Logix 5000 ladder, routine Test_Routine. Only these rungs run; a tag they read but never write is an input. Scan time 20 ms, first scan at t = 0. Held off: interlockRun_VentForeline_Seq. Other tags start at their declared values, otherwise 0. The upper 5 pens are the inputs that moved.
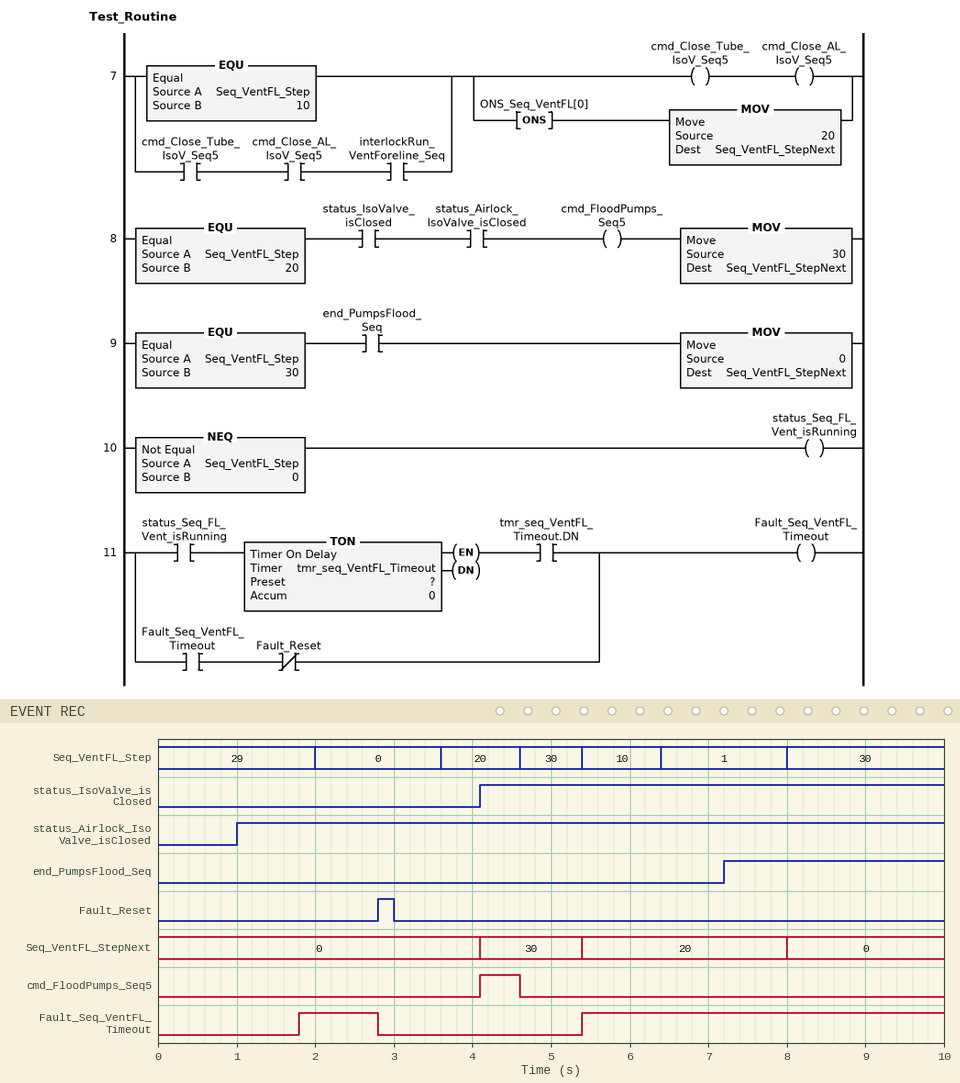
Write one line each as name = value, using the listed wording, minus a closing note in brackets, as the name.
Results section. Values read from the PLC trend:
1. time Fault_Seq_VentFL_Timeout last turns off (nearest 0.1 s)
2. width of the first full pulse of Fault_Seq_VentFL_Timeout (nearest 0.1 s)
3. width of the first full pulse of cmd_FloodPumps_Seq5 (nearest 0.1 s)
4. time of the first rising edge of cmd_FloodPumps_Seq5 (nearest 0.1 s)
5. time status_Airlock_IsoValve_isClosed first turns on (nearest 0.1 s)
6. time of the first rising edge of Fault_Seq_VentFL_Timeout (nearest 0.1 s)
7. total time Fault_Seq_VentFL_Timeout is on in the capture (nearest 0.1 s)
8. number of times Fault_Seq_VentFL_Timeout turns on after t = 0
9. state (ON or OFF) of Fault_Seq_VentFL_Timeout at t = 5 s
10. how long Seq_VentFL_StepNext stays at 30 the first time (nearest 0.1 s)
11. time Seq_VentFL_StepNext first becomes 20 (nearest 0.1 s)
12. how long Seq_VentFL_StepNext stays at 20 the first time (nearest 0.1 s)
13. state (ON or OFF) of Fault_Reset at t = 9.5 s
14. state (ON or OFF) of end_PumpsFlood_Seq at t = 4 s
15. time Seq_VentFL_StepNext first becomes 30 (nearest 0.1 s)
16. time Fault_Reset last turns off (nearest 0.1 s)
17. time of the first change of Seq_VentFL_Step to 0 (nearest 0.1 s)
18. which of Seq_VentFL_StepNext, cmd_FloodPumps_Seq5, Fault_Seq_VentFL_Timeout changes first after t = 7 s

time Fault_Seq_VentFL_Timeout last turns off = 2.8 s
width of the first full pulse of Fault_Seq_VentFL_Timeout = 1.0 s
width of the first full pulse of cmd_FloodPumps_Seq5 = 0.5 s
time of the first rising edge of cmd_FloodPumps_Seq5 = 4.1 s
time status_Airlock_IsoValve_isClosed first turns on = 1.0 s
time of the first rising edge of Fault_Seq_VentFL_Timeout = 1.8 s
total time Fault_Seq_VentFL_Timeout is on in the capture = 5.6 s
number of times Fault_Seq_VentFL_Timeout turns on after t = 0 = 2
state (ON or OFF) of Fault_Seq_VentFL_Timeout at t = 5 s = OFF
how long Seq_VentFL_StepNext stays at 30 the first time = 1.3 s
time Seq_VentFL_StepNext first becomes 20 = 5.4 s
how long Seq_VentFL_StepNext stays at 20 the first time = 2.6 s
state (ON or OFF) of Fault_Reset at t = 9.5 s = OFF
state (ON or OFF) of end_PumpsFlood_Seq at t = 4 s = OFF
time Seq_VentFL_StepNext first becomes 30 = 4.1 s
time Fault_Reset last turns off = 3.0 s
time of the first change of Seq_VentFL_Step to 0 = 2.0 s
which of Seq_VentFL_StepNext, cmd_FloodPumps_Seq5, Fault_Seq_VentFL_Timeout changes first after t = 7 s = Seq_VentFL_StepNext
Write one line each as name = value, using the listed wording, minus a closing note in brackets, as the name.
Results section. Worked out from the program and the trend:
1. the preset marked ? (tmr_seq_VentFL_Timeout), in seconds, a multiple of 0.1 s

the preset marked ? (tmr_seq_VentFL_Timeout), in seconds, a multiple of 0.1 s = 1.8 s
